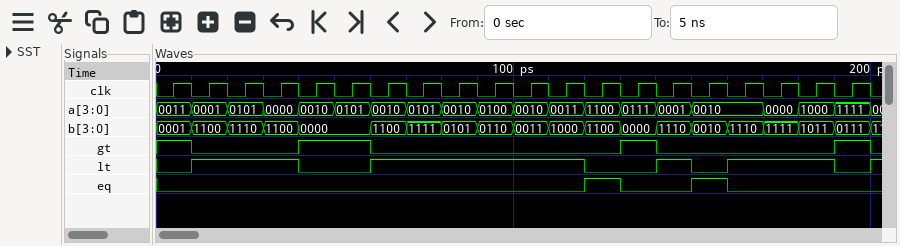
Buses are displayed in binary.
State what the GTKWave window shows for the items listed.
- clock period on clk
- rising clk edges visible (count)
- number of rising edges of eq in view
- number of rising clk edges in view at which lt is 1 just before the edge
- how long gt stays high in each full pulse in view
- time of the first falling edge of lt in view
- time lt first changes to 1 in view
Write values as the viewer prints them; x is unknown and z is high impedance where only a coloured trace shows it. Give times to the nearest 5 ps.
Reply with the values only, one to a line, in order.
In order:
10 ps
20
2
13
20 ps, 10 ps, 10 ps
40 ps
10 ps
